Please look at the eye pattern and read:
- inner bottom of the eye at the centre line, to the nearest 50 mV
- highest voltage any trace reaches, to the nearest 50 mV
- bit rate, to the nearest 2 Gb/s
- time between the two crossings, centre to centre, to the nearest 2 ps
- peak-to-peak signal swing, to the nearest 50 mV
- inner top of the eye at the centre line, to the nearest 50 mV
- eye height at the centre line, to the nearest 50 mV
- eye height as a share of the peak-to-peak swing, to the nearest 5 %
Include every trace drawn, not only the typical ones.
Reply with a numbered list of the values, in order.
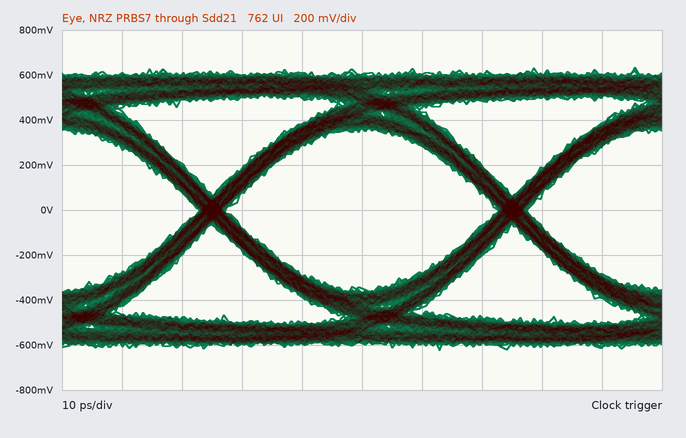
1. -350 mV
2. 650 mV
3. 20 Gb/s
4. 50 ps
5. 1.25 V
6. 350 mV
7. 700 mV
8. 55 %
